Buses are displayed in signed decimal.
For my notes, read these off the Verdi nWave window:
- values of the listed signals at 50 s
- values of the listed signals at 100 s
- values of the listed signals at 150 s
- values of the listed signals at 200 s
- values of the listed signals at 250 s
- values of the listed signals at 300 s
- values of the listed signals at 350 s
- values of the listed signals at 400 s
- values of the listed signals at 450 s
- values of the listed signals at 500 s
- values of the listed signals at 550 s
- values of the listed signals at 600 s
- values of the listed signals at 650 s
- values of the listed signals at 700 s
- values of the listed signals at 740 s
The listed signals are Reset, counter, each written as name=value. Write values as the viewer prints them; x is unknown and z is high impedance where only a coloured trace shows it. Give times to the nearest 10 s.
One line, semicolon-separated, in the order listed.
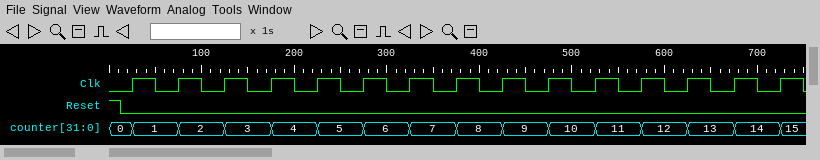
Reset=0, counter=1; Reset=0, counter=2; Reset=0, counter=3; Reset=0, counter=4; Reset=0, counter=5; Reset=0, counter=6; Reset=0, counter=7; Reset=0, counter=8; Reset=0, counter=9; Reset=0, counter=10; Reset=0, counter=11; Reset=0, counter=12; Reset=0, counter=13; Reset=0, counter=14; Reset=0, counter=15
